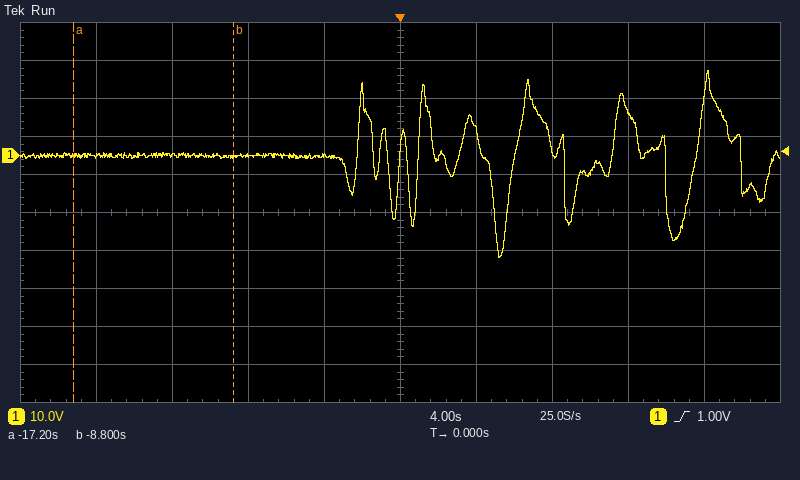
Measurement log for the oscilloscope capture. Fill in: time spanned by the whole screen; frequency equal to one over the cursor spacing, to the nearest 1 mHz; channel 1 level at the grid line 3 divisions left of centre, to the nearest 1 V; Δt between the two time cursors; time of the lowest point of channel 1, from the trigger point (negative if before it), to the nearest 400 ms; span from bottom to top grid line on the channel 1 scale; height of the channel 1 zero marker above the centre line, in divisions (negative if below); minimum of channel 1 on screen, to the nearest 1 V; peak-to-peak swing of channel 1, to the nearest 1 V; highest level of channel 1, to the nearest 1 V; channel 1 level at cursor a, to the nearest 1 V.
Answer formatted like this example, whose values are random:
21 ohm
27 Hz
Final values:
40 s
119 mHz
0 V
8.4 s
+5.2 s
100 V
+1.5 div
-27 V
49 V
22 V
0 V
